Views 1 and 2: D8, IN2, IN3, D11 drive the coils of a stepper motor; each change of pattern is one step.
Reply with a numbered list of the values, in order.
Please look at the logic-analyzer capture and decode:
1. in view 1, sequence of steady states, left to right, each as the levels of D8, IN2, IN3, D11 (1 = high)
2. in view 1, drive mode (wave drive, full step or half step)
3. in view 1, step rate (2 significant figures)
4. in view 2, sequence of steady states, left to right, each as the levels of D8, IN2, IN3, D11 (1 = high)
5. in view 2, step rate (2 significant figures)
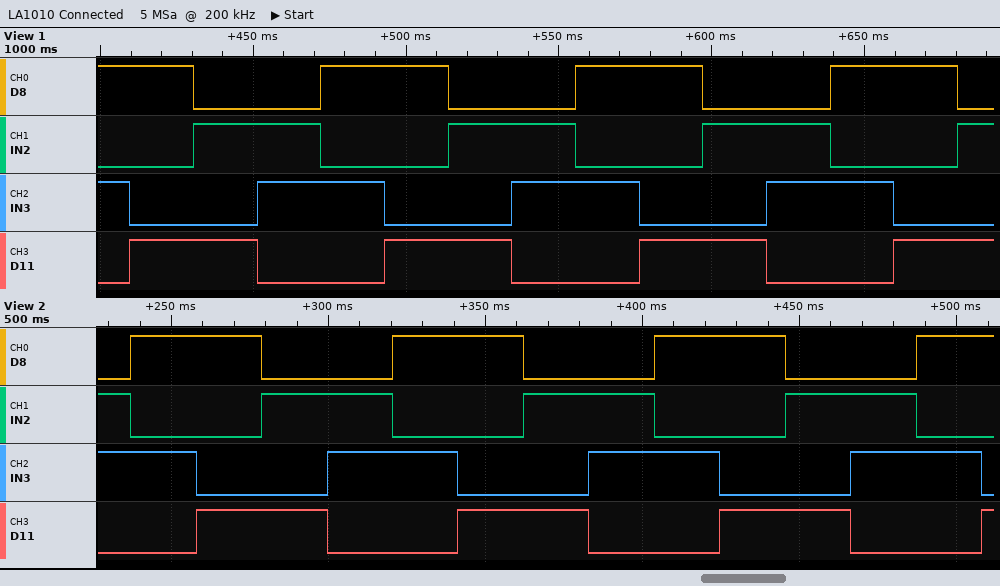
1. 1010 1001 0101 0110 1010 1001 0101 0110 1010 1001 0101 0110 1010 1001 0101
2. full step
3. 48 steps/s
4. 0110 1010 1001 0101 0110 1010 1001 0101 0110 1010 1001 0101 0110 1010 1001
5. 48 steps/s
